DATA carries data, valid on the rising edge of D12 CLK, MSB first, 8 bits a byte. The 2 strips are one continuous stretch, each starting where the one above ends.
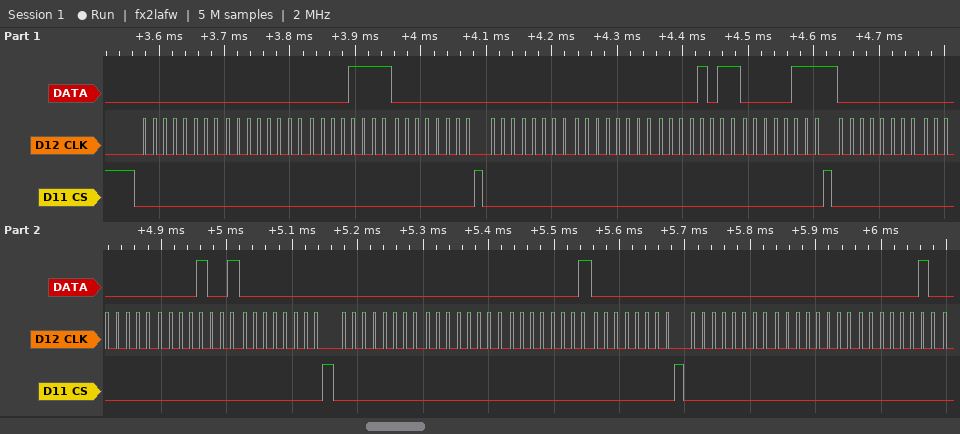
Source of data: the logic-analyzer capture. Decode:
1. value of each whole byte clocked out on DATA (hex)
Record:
0x00 0x00 0x0F 0x00 0x00 0x00 0x0B 0x07 0x00 0x00 0x09 0x00 0x00 0x00 0x01 0x00 0x00 0x00 0x02
